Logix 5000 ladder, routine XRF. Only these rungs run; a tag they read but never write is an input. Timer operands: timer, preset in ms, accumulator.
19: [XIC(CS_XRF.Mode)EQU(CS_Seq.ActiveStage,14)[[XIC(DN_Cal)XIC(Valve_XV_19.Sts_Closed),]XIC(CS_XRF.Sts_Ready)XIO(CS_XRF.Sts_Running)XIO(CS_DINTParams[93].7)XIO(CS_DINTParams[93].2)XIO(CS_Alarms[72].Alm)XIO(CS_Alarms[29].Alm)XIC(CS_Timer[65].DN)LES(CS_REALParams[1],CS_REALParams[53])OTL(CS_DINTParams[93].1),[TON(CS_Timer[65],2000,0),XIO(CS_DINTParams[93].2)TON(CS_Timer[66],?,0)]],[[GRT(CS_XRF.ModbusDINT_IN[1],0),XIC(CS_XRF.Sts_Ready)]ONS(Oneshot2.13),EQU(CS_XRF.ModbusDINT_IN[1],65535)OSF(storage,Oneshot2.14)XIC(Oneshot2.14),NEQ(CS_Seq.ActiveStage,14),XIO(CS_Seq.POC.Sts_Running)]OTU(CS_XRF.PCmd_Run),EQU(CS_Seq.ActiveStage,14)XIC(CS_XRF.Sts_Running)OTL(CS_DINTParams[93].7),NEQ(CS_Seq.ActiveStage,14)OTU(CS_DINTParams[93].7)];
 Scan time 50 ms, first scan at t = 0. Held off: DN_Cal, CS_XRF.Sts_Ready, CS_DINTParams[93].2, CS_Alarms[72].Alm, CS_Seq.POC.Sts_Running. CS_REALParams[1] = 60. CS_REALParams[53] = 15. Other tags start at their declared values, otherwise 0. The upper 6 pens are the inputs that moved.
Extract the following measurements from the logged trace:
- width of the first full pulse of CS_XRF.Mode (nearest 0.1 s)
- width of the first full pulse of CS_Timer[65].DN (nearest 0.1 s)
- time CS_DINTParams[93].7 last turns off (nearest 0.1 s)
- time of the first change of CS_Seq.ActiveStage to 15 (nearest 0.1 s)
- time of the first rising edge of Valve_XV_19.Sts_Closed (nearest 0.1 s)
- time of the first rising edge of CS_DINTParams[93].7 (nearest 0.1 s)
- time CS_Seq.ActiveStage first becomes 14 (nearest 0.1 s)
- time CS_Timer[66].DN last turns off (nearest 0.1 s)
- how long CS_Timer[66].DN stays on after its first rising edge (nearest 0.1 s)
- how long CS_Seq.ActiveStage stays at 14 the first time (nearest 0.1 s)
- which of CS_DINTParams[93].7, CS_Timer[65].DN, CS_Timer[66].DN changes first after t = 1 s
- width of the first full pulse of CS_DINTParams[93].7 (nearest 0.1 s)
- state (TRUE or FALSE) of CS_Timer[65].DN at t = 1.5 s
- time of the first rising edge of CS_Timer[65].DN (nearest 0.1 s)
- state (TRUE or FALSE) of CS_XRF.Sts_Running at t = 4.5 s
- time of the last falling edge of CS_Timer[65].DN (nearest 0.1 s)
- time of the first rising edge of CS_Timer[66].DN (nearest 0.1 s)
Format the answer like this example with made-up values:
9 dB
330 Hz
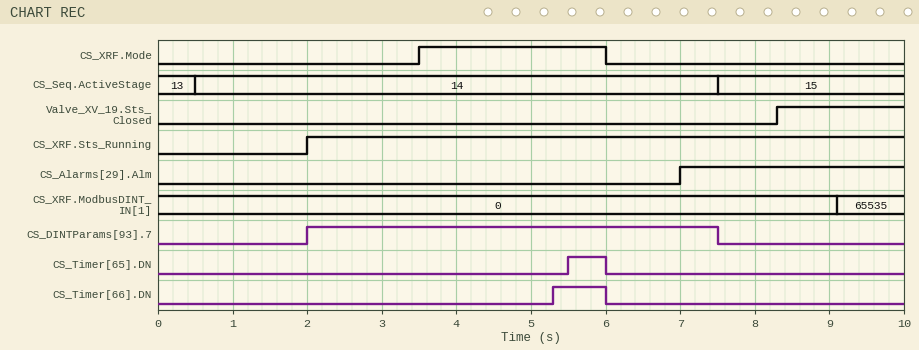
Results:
2.5 s
0.5 s
7.5 s
7.5 s
8.3 s
2.0 s
0.5 s
6.0 s
0.7 s
7.0 s
CS_DINTParams[93].7
5.5 s
FALSE
5.5 s
TRUE
6.0 s
5.3 s
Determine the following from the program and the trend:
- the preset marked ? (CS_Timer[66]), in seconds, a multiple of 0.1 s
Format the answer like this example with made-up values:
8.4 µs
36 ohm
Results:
1.8 s
